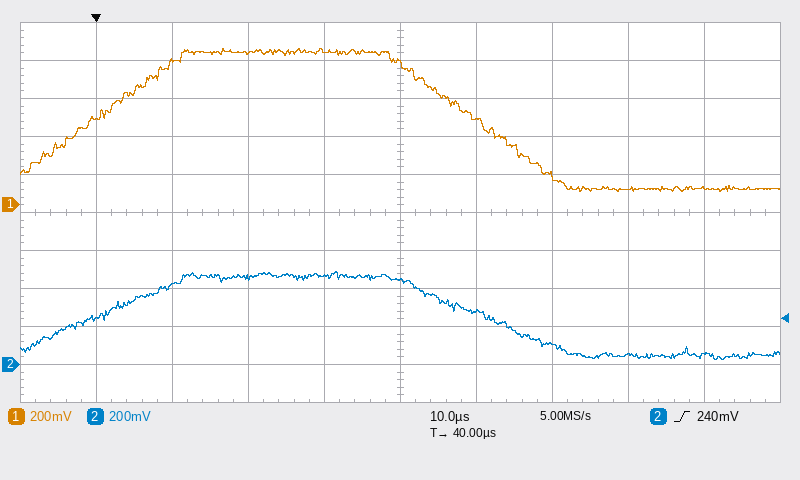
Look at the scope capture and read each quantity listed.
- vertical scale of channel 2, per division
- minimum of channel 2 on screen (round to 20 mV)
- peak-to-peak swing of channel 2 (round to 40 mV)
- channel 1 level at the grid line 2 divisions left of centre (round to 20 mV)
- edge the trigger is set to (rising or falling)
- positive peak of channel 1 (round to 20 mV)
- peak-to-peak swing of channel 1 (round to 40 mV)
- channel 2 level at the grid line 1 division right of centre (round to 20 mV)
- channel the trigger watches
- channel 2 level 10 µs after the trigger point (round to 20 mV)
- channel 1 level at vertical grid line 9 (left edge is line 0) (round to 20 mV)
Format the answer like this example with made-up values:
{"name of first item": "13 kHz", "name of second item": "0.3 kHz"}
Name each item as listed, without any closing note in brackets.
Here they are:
{"vertical scale of channel 2, per division": "200 mV", "minimum of channel 2 on screen": "20 mV", "peak-to-peak swing of channel 2": "480 mV", "channel 1 level at the grid line 2 divisions left of centre": "800 mV", "edge the trigger is set to": "rising", "positive peak of channel 1": "820 mV", "peak-to-peak swing of channel 1": "760 mV", "channel 2 level at the grid line 1 division right of centre": "280 mV", "channel the trigger watches": "channel 2", "channel 2 level 10 µs after the trigger point": "420 mV", "channel 1 level at vertical grid line 9 (left edge is line 0)": "80 mV"}
